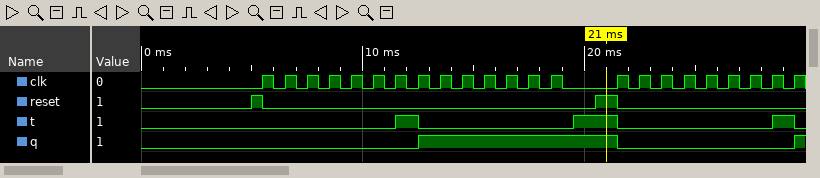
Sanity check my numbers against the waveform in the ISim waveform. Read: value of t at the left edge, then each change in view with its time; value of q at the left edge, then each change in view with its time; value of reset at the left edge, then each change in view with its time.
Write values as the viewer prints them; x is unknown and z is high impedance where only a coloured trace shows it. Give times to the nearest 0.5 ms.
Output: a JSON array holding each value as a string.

["0, 1 at 11.5 ms, 0 at 12.5 ms, 1 at 19.5 ms, 0 at 21.5 ms, 1 at 28.5 ms, 0 at 29.5 ms", "0, 1 at 12.5 ms, 0 at 21.5 ms, 1 at 29.5 ms", "0, 1 at 5 ms, 0 at 5.5 ms, 1 at 20.5 ms, 0 at 21.5 ms"]
